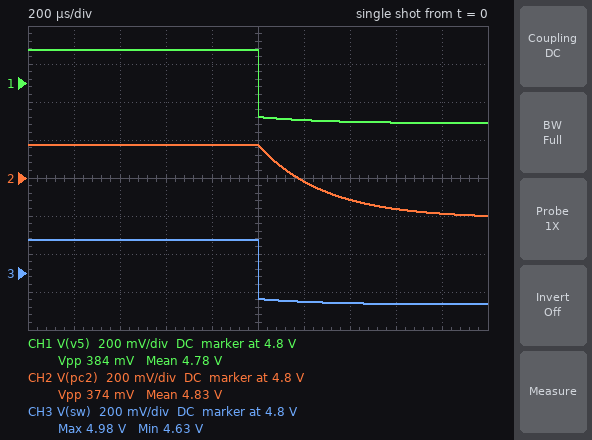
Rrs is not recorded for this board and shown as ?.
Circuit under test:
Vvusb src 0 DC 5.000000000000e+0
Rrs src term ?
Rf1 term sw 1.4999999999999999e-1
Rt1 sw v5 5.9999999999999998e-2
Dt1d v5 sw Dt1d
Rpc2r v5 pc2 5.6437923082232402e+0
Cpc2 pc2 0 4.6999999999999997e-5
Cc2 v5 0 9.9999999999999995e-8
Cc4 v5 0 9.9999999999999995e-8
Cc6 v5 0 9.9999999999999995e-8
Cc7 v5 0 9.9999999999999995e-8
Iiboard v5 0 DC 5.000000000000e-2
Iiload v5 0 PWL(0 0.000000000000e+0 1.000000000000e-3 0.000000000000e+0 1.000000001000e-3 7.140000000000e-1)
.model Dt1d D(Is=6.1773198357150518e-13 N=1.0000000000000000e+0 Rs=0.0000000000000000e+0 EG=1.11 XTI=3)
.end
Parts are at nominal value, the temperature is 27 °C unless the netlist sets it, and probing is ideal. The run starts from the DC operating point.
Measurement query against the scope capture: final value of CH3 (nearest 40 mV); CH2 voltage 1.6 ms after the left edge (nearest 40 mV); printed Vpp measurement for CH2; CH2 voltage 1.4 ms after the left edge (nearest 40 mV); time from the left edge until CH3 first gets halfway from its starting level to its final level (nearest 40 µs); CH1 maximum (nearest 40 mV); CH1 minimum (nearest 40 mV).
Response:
4.64 V
4.64 V
374 mV
4.68 V
1.00 ms
4.96 V
4.60 V
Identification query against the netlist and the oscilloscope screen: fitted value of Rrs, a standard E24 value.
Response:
0.33 Ω
